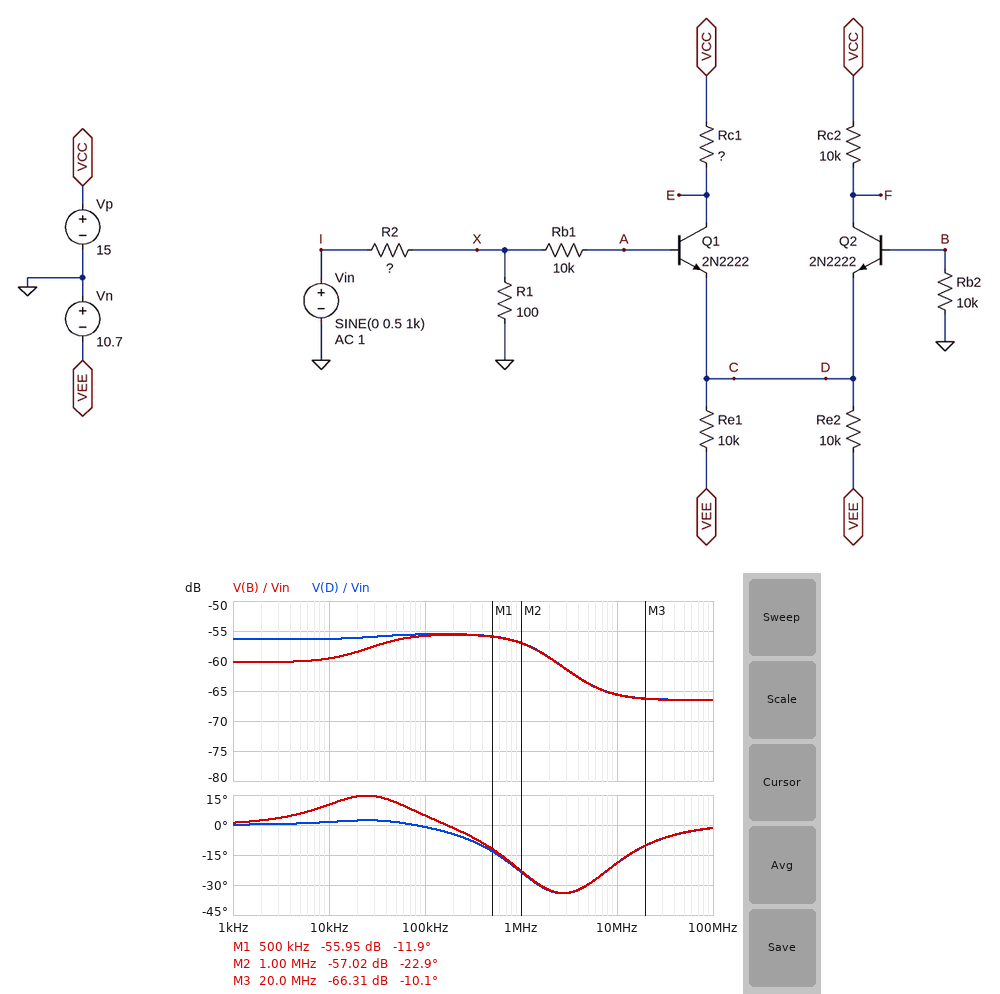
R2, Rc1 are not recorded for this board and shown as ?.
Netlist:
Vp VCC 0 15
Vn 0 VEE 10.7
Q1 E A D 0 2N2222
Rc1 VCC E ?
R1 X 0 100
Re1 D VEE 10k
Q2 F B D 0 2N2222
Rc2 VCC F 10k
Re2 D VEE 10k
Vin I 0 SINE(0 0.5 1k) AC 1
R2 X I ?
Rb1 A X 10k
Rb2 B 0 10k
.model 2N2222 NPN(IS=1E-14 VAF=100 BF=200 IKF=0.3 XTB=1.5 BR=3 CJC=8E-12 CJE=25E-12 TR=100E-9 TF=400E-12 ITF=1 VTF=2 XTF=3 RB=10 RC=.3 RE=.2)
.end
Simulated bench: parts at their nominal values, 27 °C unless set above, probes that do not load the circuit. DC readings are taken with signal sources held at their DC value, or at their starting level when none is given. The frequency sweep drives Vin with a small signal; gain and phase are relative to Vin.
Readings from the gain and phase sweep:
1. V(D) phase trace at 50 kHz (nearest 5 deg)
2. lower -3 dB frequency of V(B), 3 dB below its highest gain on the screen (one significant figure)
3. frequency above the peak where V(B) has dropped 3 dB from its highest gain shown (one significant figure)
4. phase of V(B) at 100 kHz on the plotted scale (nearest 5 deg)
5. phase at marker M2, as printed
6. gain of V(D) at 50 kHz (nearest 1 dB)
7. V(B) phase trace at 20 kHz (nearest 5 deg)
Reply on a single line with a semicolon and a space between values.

0 deg; 20 kHz; 2 MHz; 5 deg; -22.9 deg; -56 dB; 15 deg
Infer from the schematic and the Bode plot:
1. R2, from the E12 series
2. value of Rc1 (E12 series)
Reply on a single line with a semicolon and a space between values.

33 kΩ; 8.2 kΩ
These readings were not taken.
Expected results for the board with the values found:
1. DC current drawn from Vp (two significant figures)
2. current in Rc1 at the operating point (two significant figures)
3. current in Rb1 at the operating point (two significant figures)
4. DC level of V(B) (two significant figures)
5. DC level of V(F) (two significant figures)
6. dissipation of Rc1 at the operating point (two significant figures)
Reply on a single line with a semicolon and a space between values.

2.0 mA; 1.0 mA; 4.7 µA; -47 mV; 5.1 V; 8.2 mW
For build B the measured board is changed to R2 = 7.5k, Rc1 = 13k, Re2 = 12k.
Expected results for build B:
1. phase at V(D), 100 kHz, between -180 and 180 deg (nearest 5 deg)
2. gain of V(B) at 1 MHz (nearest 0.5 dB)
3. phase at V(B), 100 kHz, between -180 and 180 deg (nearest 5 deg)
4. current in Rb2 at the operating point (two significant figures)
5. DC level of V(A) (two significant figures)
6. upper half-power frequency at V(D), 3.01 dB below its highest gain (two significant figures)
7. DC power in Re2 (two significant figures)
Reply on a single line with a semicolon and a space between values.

-5 deg; -47.5 dB; 0 deg; 4.4 µA; -44 mV; 810 kHz; 8.3 mW
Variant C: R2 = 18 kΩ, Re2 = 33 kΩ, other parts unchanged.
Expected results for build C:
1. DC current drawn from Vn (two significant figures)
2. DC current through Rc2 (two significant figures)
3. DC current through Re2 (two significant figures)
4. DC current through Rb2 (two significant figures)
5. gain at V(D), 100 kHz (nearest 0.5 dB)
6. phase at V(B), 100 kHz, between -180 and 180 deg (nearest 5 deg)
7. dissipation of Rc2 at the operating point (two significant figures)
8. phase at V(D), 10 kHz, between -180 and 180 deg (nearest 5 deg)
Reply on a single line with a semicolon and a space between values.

1.3 mA; 650 µA; 300 µA; 3.0 µA; -50.5 dB; 10 deg; 4.2 mW; 0 deg
